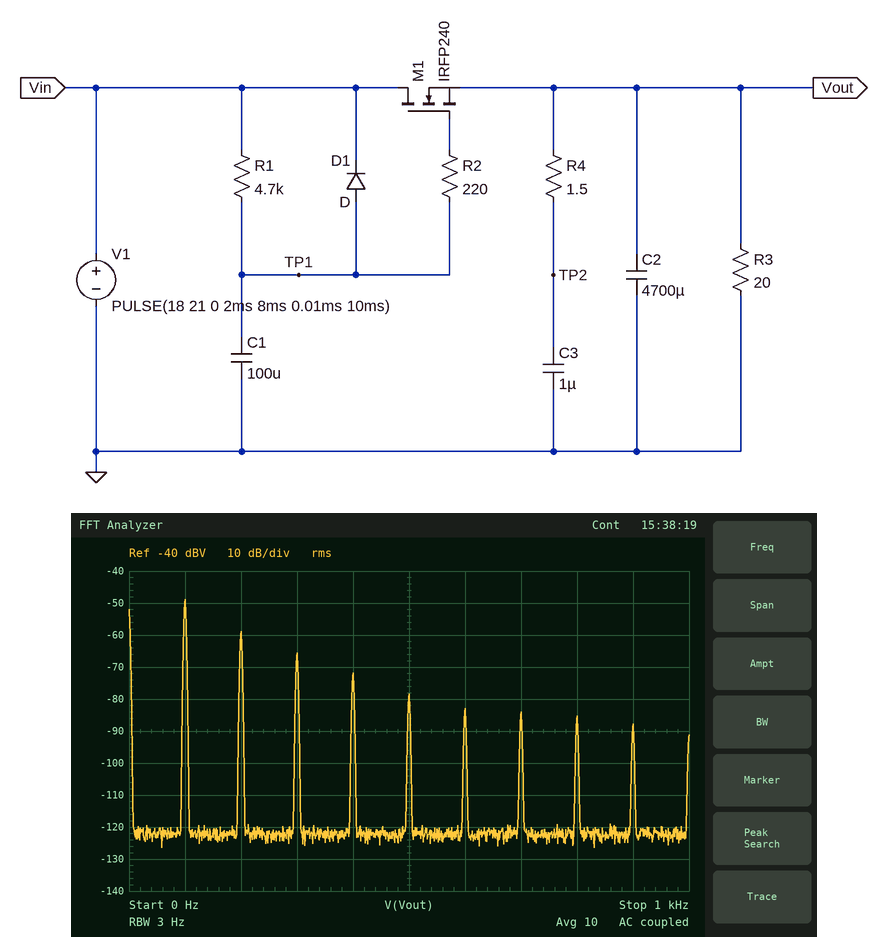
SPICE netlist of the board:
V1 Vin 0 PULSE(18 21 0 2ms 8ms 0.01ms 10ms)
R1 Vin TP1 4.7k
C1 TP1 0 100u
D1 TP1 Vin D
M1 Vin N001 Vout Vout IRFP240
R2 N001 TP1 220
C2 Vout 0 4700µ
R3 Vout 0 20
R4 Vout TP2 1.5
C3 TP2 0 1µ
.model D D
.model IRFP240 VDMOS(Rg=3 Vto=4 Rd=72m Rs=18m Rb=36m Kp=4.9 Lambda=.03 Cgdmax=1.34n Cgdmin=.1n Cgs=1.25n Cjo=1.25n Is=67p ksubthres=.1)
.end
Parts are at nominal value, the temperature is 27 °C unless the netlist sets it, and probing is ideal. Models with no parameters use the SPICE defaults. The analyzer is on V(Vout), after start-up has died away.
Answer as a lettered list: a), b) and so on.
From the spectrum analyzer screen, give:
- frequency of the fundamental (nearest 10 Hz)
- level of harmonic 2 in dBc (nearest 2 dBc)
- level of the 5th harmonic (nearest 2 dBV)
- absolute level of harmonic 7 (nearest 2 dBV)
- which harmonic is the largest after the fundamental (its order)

a) 100 Hz
b) -10 dBc
c) -78 dBV
d) -84 dBV
e) 2
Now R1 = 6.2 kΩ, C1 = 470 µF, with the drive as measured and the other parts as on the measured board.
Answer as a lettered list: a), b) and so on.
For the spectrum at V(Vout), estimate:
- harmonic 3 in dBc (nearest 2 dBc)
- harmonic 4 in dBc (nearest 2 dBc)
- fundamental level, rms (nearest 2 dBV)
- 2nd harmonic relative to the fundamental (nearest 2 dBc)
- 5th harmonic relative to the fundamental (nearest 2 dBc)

a) -20 dBc
b) -30 dBc
c) -50 dBV
d) -12 dBc
e) -44 dBc
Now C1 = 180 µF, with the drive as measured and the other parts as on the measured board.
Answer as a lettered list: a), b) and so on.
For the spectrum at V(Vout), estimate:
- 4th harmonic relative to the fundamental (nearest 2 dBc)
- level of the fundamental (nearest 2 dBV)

a) -24 dBc
b) -50 dBV
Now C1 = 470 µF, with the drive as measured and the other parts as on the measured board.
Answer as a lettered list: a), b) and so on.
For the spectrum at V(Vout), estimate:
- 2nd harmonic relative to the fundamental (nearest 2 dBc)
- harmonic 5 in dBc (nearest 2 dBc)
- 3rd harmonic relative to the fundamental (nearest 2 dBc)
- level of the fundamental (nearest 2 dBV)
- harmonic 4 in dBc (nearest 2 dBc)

a) -12 dBc
b) -42 dBc
c) -20 dBc
d) -50 dBV
e) -30 dBc
